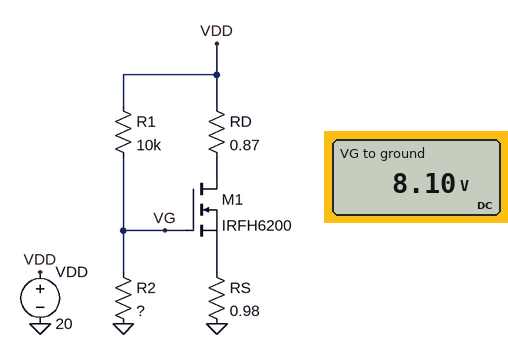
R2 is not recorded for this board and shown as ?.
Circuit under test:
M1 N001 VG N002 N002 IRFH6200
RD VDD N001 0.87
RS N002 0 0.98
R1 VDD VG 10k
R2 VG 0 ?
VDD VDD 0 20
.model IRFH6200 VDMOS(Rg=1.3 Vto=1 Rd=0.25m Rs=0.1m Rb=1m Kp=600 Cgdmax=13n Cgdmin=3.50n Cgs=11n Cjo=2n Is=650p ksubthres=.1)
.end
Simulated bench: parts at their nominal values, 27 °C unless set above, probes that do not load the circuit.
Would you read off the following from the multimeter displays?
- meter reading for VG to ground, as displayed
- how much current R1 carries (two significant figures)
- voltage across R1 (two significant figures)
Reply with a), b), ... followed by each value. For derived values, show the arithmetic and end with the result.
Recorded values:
a) 8.10 V
b) (20 V - 8.1 V) / 10 kΩ = 1.2 mA
c) 20 V - 8.1 V = 12 V
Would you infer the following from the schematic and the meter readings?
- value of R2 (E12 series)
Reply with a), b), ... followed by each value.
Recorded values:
a) 6.8 kΩ
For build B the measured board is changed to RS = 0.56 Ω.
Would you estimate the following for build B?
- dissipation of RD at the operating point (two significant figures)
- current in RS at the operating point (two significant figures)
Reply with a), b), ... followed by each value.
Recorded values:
a) 130 W
b) 12 A
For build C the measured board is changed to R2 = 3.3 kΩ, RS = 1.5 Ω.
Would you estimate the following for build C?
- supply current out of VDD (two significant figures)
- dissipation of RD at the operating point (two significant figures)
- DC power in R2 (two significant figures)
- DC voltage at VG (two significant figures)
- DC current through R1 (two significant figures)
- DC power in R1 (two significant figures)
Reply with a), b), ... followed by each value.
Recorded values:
a) 2.6 A
b) 5.9 W
c) 7.5 mW
d) 5.0 V
e) 1.5 mA
f) 23 mW
